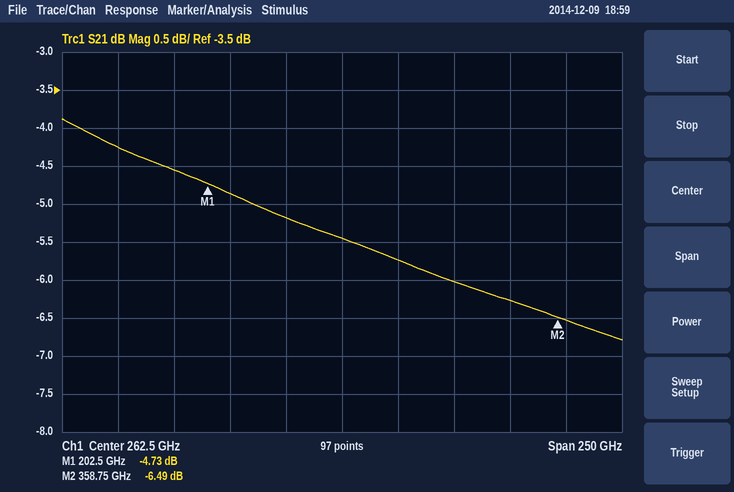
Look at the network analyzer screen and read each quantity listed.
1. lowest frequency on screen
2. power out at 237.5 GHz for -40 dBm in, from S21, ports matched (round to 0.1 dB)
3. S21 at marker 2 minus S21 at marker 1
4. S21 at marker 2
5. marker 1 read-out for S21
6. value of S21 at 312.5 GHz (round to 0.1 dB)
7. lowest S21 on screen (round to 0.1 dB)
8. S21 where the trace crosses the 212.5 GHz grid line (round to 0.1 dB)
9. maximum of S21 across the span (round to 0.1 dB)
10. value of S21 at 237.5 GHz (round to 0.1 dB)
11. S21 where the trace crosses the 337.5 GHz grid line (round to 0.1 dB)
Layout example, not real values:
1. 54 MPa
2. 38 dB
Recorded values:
1. 137.5 GHz
2. -45.2 dBm
3. -1.76 dB
4. -6.49 dB
5. -4.73 dB
6. -6.0 dB
7. -6.8 dB
8. -4.9 dB
9. -3.9 dB
10. -5.2 dB
11. -6.3 dB
